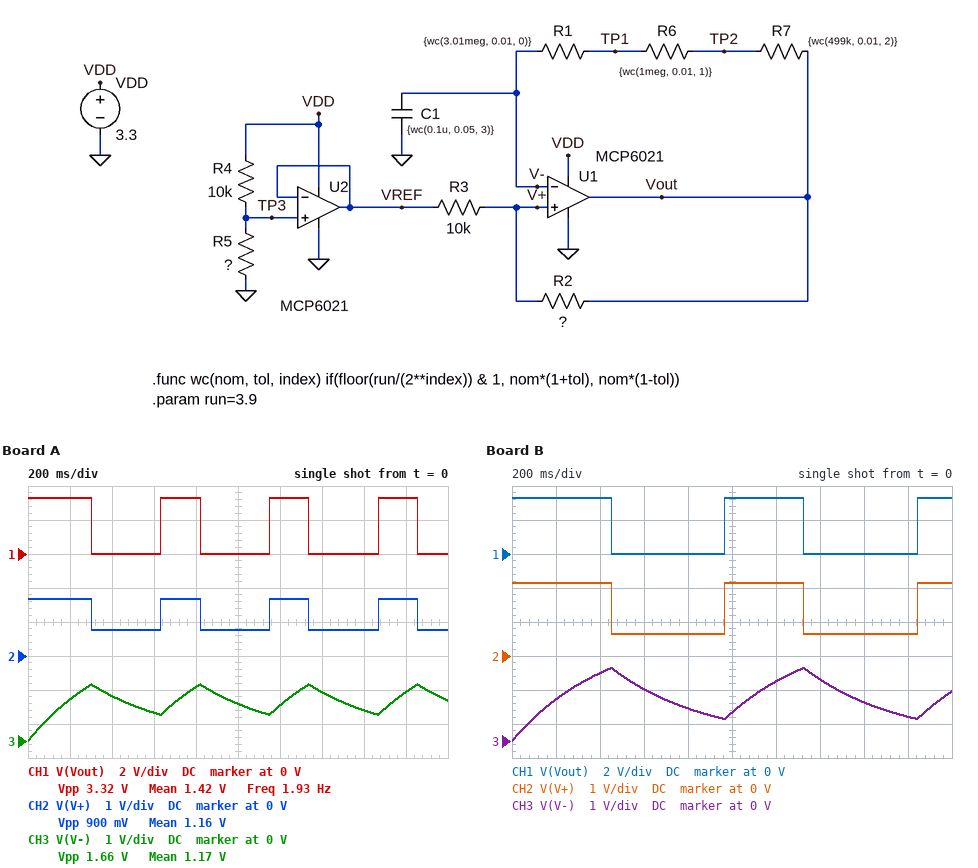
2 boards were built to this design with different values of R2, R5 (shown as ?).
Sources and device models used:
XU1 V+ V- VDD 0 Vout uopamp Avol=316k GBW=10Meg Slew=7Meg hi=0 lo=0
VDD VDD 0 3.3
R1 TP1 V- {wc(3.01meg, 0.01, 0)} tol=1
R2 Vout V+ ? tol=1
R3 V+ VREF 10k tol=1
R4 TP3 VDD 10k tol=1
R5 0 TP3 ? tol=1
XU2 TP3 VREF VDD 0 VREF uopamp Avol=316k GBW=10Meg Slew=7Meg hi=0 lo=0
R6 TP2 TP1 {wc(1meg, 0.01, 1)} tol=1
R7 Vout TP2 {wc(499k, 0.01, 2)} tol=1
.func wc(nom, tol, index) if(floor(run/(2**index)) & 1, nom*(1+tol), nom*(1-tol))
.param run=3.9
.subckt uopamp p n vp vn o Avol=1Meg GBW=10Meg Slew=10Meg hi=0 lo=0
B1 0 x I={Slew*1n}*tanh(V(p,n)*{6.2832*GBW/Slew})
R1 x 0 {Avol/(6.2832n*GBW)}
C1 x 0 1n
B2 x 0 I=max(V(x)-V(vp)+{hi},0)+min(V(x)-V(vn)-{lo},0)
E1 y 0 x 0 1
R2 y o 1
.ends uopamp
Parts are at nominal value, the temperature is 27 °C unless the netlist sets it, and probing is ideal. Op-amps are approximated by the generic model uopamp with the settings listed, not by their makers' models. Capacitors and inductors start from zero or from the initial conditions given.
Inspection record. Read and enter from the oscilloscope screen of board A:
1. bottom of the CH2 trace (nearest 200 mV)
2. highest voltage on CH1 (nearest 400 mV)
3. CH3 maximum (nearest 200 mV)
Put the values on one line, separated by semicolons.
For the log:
800 mV; 3.2 V; 1.6 V
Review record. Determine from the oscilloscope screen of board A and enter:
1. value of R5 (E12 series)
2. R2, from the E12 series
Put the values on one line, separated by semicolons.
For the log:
4.7 kΩ; 27 kΩ
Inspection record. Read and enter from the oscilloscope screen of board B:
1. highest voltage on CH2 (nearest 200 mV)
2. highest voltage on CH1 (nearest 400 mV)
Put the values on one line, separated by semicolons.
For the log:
2.2 V; 3.2 V
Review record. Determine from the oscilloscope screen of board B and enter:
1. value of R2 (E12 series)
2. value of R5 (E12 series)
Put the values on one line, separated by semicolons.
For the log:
12 kΩ; 5.6 kΩ
